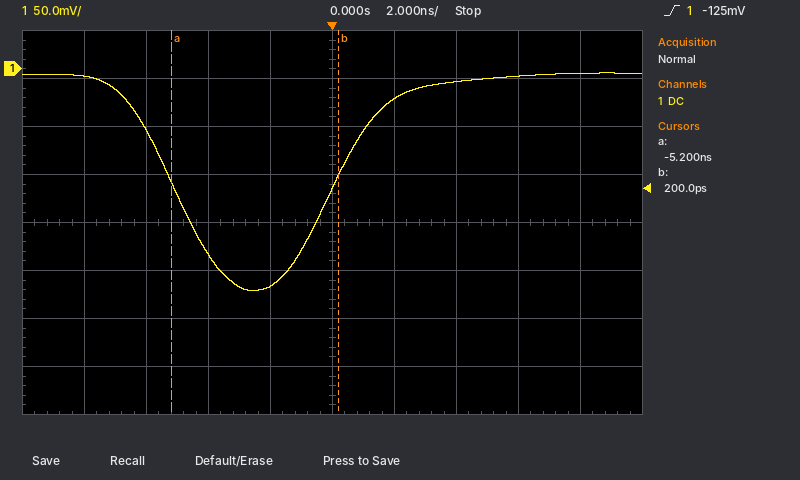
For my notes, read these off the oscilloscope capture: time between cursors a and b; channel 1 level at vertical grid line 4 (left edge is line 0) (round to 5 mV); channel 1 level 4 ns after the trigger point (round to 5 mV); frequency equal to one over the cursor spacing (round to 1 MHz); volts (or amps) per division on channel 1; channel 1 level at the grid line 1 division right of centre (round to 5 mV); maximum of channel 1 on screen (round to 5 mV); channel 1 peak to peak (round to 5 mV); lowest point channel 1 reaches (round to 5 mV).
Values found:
5.4 ns
-225 mV
-15 mV
185 MHz
50 mV
-30 mV
-5 mV
225 mV
-230 mV
